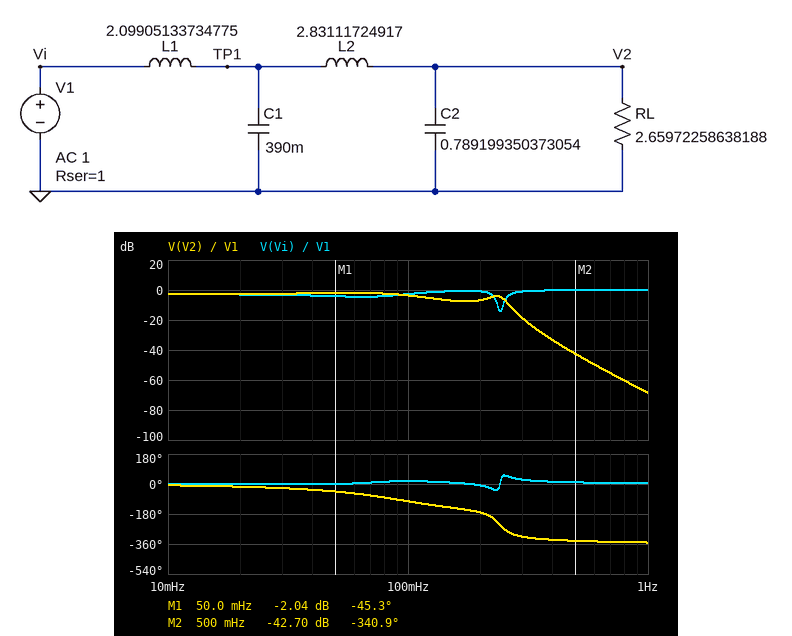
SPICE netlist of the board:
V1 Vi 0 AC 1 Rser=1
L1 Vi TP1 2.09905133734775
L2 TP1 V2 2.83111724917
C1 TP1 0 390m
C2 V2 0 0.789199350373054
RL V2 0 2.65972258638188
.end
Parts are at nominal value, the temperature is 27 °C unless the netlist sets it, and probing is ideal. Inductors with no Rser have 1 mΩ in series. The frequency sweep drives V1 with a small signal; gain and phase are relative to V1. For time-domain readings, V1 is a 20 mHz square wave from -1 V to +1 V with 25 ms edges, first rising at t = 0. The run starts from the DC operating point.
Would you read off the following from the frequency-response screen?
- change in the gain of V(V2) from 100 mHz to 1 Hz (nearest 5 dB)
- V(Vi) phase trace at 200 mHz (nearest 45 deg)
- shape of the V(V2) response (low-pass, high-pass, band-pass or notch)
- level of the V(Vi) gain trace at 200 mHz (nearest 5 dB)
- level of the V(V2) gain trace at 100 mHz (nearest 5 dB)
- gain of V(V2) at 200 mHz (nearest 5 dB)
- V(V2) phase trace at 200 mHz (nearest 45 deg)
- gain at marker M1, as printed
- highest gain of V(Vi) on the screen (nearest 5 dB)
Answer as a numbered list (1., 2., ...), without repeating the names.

1. -65 dB
2. 0 deg
3. low-pass
4. 0 dB
5. -5 dB
6. -5 dB
7. -180 deg
8. -2.04 dB
9. 0 dB
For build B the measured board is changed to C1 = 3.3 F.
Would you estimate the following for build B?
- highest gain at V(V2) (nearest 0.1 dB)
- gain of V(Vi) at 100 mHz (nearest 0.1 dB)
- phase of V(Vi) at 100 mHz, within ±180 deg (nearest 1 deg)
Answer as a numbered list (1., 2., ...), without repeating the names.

1. -2.6 dB
2. -4.7 dB
3. 40 deg
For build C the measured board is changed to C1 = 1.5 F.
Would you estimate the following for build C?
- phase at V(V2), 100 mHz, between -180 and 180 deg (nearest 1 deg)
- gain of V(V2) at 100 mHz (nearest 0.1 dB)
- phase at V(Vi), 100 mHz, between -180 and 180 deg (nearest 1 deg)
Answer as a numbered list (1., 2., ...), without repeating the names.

1. -135 deg
2. -2.5 dB
3. 19 deg
